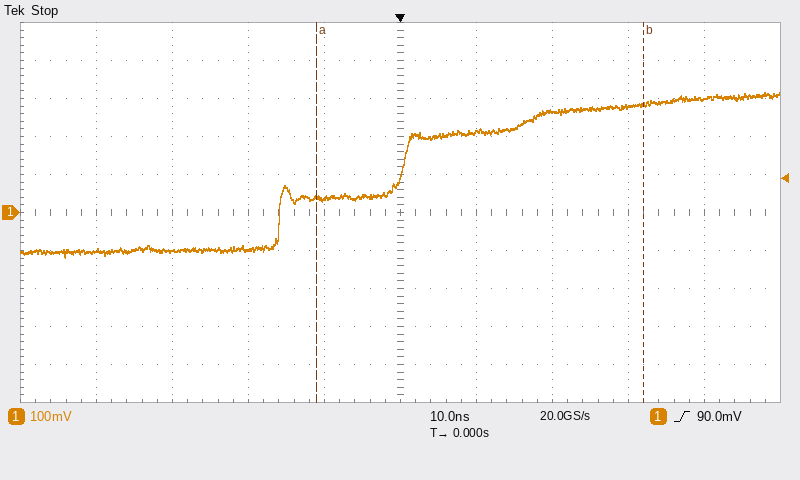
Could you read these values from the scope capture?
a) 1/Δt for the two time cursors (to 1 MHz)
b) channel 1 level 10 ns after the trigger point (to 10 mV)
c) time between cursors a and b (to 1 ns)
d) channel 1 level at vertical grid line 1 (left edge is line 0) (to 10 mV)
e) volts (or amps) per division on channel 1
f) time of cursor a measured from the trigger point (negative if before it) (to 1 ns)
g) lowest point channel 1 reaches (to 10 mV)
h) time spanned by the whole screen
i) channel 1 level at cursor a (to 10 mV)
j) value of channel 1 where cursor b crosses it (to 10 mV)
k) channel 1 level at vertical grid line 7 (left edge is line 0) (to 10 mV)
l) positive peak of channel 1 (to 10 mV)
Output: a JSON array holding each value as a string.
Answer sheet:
["23 MHz", "210 mV", "43 ns", "-100 mV", "100 mV", "-11 ns", "-120 mV", "100 ns", "40 mV", "280 mV", "270 mV", "320 mV"]
